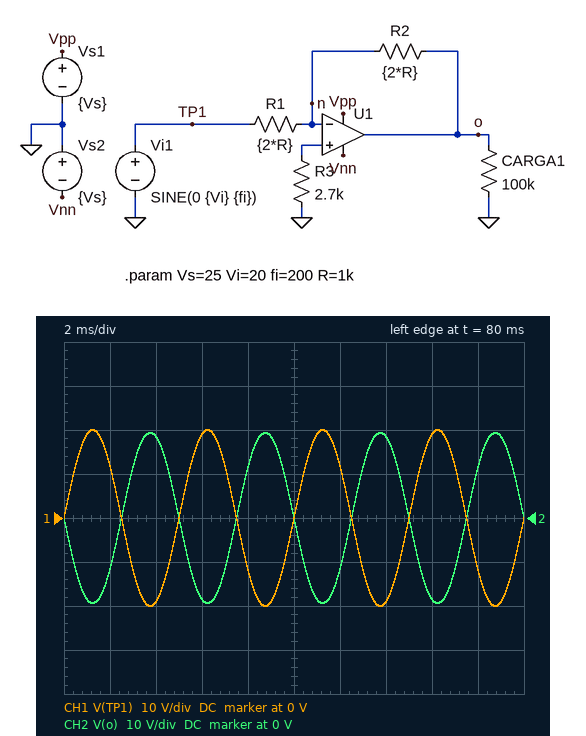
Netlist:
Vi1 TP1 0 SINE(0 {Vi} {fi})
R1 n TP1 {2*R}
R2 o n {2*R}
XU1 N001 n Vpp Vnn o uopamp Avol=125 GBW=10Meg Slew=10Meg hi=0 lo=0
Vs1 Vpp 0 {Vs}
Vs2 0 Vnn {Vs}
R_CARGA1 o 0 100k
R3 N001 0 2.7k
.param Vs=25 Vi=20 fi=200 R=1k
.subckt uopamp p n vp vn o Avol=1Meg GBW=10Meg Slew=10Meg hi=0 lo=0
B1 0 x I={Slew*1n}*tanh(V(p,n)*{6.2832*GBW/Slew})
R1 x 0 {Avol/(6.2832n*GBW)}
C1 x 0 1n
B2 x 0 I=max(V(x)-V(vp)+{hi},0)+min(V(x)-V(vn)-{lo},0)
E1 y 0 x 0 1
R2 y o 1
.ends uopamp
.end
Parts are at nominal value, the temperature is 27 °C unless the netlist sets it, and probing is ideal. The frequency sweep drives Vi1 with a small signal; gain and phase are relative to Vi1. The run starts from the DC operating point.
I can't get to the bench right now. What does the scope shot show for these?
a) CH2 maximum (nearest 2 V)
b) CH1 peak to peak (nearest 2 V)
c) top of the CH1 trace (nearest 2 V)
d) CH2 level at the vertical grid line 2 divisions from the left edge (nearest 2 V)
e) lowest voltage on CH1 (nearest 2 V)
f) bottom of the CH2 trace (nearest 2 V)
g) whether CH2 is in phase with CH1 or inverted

20 V
40 V
20 V
18 V
-20 V
-20 V
inverted
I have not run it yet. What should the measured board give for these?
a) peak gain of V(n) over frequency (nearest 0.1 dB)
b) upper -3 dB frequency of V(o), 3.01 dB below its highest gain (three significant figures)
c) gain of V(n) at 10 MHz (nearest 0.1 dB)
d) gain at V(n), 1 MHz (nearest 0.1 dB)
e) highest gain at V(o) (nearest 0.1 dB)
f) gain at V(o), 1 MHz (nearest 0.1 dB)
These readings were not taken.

-6.0 dB
5.08 MHz
-7.0 dB
-20.3 dB
-0.1 dB
-0.3 dB
